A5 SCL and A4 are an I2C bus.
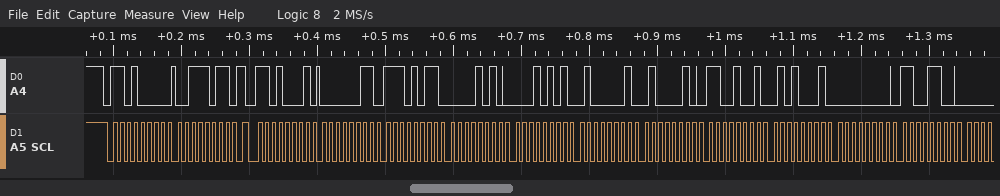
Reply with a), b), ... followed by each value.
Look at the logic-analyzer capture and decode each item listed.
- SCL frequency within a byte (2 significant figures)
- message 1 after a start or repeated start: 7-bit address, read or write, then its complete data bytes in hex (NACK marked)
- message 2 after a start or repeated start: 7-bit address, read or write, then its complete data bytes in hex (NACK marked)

a) 100 kHz
b) 0x68 write: 3B
c) 0x68 read: 03 EB 0A 15 41 42 C9 51 00 CC
